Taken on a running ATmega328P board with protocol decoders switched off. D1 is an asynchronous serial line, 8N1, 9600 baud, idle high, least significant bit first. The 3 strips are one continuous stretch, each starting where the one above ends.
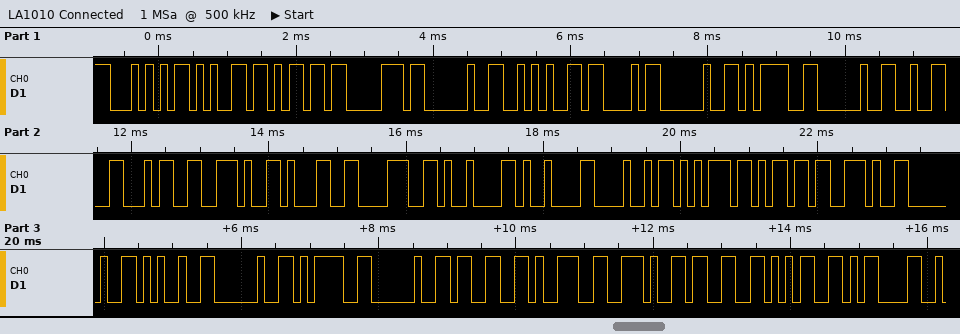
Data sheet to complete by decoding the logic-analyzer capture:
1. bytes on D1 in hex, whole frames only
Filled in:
0x54 0x65 0x6D 0x70 0x20 0x2A 0x43 0x20 0x3D 0x20 0x32 0x34 0x2E 0x31 0x38 0x09 0x09 0x48 0x75 0x6D 0x2E 0x20 0x25 0x20 0x3D 0x20 0x33 0x39 0x2E 0x33 0x35 0x0D
